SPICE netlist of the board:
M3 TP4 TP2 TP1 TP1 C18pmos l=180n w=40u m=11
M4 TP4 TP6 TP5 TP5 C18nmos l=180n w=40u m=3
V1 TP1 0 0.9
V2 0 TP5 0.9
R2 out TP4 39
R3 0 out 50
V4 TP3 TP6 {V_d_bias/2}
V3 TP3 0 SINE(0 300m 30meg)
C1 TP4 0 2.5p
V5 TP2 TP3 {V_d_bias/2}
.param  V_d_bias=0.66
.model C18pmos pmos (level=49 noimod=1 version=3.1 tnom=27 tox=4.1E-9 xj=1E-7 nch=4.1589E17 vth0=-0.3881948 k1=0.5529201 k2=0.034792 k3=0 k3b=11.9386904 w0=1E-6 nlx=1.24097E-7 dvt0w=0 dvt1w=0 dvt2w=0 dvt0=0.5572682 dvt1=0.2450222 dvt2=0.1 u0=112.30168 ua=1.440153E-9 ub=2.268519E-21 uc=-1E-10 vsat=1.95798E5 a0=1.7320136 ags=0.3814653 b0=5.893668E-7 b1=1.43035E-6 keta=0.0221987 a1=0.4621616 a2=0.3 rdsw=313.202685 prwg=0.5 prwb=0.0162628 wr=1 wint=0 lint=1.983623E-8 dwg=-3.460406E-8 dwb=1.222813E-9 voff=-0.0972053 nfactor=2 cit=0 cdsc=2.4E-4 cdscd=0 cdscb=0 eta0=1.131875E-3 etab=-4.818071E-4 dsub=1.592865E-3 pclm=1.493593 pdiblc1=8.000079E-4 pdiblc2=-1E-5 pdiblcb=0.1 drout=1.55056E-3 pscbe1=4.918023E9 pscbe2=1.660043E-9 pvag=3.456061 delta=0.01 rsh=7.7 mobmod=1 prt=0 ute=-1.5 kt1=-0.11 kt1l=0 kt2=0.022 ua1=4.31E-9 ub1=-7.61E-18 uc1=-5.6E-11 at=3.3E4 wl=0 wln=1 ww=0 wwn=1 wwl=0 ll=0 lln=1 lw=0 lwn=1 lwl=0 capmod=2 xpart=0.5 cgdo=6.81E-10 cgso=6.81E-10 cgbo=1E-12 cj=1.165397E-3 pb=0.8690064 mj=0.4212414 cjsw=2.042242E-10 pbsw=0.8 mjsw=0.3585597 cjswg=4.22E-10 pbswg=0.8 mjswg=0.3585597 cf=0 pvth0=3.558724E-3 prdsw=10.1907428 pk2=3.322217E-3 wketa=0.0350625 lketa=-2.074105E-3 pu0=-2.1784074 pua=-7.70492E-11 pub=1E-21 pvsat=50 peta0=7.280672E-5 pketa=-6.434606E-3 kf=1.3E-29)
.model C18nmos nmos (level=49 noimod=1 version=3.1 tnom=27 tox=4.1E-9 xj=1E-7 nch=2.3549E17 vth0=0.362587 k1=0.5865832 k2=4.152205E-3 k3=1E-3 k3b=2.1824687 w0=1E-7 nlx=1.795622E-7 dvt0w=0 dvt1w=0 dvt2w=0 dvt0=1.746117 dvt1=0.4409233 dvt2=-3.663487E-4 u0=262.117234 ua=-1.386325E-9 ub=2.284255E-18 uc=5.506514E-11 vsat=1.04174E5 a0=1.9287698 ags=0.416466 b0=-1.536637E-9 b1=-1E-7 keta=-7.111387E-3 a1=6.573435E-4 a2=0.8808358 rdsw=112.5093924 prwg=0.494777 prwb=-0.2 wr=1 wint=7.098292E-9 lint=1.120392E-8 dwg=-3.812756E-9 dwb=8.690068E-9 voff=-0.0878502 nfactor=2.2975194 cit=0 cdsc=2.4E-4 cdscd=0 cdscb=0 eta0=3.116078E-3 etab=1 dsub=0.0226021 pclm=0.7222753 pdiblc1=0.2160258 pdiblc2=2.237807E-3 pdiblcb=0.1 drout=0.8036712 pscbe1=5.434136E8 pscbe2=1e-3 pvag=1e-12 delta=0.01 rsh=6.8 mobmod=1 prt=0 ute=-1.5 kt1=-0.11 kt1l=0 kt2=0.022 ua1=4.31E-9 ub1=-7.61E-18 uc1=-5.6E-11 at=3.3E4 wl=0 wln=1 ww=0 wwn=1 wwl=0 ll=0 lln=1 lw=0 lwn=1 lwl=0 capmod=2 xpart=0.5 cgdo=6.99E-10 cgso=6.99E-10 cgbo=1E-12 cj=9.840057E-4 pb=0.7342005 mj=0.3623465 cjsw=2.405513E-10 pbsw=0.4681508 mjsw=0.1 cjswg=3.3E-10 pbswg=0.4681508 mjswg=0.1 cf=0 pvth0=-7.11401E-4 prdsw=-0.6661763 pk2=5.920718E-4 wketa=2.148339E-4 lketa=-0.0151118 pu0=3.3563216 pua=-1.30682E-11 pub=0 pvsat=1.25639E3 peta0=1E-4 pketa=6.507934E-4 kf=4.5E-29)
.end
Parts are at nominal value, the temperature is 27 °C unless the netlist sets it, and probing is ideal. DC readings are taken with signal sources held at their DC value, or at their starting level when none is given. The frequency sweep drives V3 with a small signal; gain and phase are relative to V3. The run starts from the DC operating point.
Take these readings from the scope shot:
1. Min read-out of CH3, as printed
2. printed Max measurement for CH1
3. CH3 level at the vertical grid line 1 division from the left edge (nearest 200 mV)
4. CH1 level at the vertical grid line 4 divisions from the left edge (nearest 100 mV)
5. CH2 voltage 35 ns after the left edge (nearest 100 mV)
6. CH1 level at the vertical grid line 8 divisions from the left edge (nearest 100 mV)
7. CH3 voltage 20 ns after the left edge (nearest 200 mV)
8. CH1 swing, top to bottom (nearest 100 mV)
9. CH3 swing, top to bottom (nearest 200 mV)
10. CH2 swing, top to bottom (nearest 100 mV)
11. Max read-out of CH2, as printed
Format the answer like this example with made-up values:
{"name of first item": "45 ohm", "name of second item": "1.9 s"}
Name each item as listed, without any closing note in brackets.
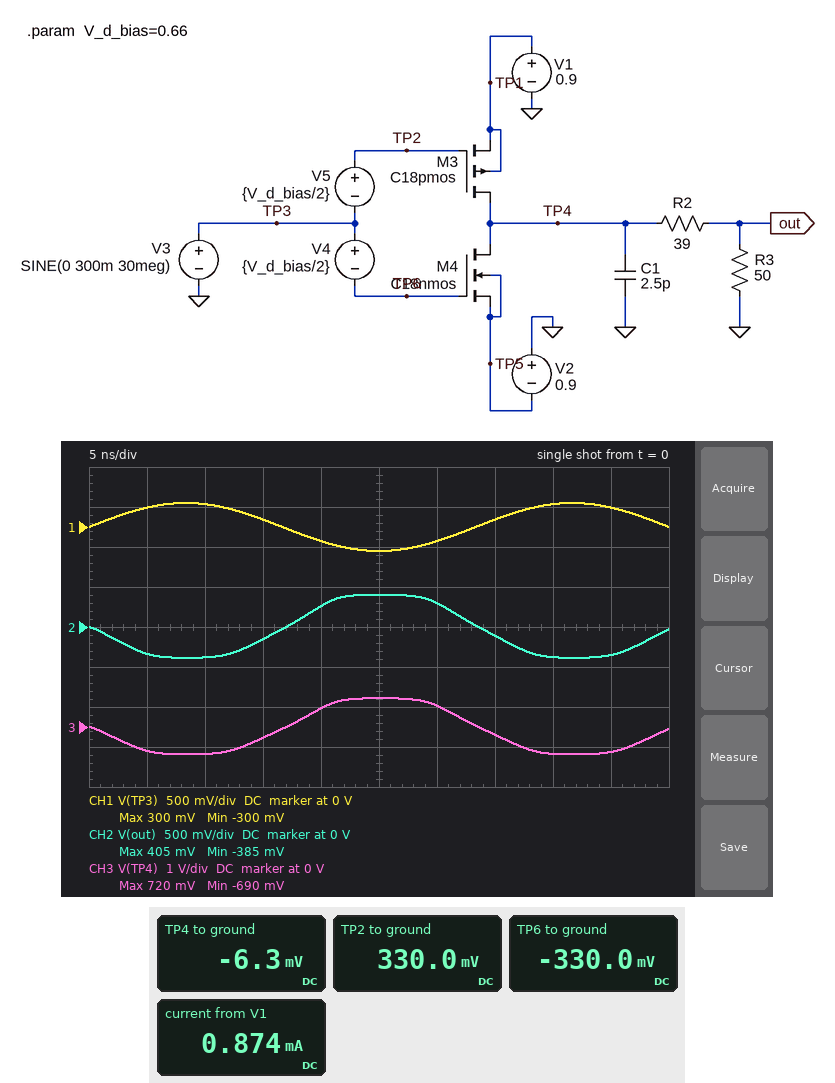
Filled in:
{"Min read-out of CH3, as printed": "-690 mV", "printed Max measurement for CH1": "300 mV", "CH3 level at the vertical grid line 1 division from the left edge": "-600 mV", "CH1 level at the vertical grid line 4 divisions from the left edge": "-200 mV", "CH2 voltage 35 ns after the left edge": "-100 mV", "CH1 level at the vertical grid line 8 divisions from the left edge": "300 mV", "CH3 voltage 20 ns after the left edge": "400 mV", "CH1 swing, top to bottom": "600 mV", "CH3 swing, top to bottom": "1.4 V", "CH2 swing, top to bottom": "800 mV", "Max read-out of CH2, as printed": "405 mV"}
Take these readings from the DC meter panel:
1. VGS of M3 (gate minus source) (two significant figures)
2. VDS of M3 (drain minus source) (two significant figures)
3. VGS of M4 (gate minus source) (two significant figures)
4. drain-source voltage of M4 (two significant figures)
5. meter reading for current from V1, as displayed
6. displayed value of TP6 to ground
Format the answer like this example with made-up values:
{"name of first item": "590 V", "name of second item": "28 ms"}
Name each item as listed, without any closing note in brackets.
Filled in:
{"VGS of M3 (gate minus source)": "-570 mV", "VDS of M3 (drain minus source)": "-910 mV", "VGS of M4 (gate minus source)": "570 mV", "drain-source voltage of M4": "890 mV", "meter reading for current from V1, as displayed": "0.874 mA", "displayed value of TP6 to ground": "-330.0 mV"}
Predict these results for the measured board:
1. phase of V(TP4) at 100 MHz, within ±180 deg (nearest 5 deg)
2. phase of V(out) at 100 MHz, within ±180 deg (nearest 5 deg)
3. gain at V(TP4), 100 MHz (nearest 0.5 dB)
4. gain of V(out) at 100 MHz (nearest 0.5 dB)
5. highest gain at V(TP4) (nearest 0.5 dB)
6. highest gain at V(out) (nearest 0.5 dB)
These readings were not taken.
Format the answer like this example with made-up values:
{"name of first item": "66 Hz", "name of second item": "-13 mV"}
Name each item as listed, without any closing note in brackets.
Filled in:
{"phase of V(TP4) at 100 MHz, within ±180 deg": "170 deg", "phase of V(out) at 100 MHz, within ±180 deg": "170 deg", "gain at V(TP4), 100 MHz": "7.5 dB", "gain of V(out) at 100 MHz": "2.5 dB", "highest gain at V(TP4)": "7.5 dB", "highest gain at V(out)": "2.5 dB"}
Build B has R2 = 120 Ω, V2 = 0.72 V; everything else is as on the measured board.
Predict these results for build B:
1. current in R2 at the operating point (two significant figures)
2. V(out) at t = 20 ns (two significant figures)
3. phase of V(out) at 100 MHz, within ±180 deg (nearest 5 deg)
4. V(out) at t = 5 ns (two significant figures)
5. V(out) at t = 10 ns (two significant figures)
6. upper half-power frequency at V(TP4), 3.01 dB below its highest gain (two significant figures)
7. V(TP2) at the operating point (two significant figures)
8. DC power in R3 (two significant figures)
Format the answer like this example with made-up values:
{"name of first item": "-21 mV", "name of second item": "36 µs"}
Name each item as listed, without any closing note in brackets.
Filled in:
{"current in R2 at the operating point": "830 µA", "V(out) at t = 20 ns": "210 mV", "phase of V(out) at 100 MHz, within ±180 deg": "160 deg", "V(out) at t = 5 ns": "-77 mV", "V(out) at t = 10 ns": "-140 mV", "upper half-power frequency at V(TP4), 3.01 dB below its highest gain": "320 MHz", "V(TP2) at the operating point": "330 mV", "DC power in R3": "34 µW"}
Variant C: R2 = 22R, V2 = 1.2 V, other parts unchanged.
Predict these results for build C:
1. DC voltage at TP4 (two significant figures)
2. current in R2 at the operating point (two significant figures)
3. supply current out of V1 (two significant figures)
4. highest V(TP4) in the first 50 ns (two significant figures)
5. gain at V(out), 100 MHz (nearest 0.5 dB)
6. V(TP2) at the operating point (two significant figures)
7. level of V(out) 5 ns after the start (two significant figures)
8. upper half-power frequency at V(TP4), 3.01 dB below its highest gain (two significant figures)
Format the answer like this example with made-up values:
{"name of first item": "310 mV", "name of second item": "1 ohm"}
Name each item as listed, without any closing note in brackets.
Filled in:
{"DC voltage at TP4": "-630 mV", "current in R2 at the operating point": "8.7 mA", "supply current out of V1": "950 µA", "highest V(TP4) in the first 50 ns": "630 mV", "gain at V(out), 100 MHz": "7.5 dB", "V(TP2) at the operating point": "330 mV", "level of V(out) 5 ns after the start": "-670 mV", "upper half-power frequency at V(TP4), 3.01 dB below its highest gain": "820 MHz"}
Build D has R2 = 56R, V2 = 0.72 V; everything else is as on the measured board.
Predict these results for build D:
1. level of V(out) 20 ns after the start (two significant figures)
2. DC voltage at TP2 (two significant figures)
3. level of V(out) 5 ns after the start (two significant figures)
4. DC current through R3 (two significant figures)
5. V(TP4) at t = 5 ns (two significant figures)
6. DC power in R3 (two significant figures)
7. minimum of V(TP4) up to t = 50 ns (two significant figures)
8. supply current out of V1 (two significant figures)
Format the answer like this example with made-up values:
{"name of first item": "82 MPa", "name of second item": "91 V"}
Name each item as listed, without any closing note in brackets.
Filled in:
{"level of V(out) 20 ns after the start": "250 mV", "DC voltage at TP2": "330 mV", "level of V(out) 5 ns after the start": "-85 mV", "DC current through R3": "840 µA", "V(TP4) at t = 5 ns": "-180 mV", "DC power in R3": "35 µW", "minimum of V(TP4) up to t = 50 ns": "-350 mV", "supply current out of V1": "860 µA"}
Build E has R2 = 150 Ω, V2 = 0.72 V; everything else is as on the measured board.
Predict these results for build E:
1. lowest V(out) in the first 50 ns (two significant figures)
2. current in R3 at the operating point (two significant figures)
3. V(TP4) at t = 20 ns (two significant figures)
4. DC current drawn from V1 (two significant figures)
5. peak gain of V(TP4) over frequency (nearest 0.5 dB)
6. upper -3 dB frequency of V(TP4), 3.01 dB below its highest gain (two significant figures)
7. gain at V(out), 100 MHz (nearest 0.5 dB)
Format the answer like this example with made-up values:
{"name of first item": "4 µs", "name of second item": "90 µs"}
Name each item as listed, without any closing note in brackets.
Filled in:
{"lowest V(out) in the first 50 ns": "-140 mV", "current in R3 at the operating point": "820 µA", "V(TP4) at t = 20 ns": "770 mV", "DC current drawn from V1": "850 µA", "peak gain of V(TP4) over frequency": "9.0 dB", "upper -3 dB frequency of V(TP4), 3.01 dB below its highest gain": "270 MHz", "gain at V(out), 100 MHz": "-3.5 dB"}
